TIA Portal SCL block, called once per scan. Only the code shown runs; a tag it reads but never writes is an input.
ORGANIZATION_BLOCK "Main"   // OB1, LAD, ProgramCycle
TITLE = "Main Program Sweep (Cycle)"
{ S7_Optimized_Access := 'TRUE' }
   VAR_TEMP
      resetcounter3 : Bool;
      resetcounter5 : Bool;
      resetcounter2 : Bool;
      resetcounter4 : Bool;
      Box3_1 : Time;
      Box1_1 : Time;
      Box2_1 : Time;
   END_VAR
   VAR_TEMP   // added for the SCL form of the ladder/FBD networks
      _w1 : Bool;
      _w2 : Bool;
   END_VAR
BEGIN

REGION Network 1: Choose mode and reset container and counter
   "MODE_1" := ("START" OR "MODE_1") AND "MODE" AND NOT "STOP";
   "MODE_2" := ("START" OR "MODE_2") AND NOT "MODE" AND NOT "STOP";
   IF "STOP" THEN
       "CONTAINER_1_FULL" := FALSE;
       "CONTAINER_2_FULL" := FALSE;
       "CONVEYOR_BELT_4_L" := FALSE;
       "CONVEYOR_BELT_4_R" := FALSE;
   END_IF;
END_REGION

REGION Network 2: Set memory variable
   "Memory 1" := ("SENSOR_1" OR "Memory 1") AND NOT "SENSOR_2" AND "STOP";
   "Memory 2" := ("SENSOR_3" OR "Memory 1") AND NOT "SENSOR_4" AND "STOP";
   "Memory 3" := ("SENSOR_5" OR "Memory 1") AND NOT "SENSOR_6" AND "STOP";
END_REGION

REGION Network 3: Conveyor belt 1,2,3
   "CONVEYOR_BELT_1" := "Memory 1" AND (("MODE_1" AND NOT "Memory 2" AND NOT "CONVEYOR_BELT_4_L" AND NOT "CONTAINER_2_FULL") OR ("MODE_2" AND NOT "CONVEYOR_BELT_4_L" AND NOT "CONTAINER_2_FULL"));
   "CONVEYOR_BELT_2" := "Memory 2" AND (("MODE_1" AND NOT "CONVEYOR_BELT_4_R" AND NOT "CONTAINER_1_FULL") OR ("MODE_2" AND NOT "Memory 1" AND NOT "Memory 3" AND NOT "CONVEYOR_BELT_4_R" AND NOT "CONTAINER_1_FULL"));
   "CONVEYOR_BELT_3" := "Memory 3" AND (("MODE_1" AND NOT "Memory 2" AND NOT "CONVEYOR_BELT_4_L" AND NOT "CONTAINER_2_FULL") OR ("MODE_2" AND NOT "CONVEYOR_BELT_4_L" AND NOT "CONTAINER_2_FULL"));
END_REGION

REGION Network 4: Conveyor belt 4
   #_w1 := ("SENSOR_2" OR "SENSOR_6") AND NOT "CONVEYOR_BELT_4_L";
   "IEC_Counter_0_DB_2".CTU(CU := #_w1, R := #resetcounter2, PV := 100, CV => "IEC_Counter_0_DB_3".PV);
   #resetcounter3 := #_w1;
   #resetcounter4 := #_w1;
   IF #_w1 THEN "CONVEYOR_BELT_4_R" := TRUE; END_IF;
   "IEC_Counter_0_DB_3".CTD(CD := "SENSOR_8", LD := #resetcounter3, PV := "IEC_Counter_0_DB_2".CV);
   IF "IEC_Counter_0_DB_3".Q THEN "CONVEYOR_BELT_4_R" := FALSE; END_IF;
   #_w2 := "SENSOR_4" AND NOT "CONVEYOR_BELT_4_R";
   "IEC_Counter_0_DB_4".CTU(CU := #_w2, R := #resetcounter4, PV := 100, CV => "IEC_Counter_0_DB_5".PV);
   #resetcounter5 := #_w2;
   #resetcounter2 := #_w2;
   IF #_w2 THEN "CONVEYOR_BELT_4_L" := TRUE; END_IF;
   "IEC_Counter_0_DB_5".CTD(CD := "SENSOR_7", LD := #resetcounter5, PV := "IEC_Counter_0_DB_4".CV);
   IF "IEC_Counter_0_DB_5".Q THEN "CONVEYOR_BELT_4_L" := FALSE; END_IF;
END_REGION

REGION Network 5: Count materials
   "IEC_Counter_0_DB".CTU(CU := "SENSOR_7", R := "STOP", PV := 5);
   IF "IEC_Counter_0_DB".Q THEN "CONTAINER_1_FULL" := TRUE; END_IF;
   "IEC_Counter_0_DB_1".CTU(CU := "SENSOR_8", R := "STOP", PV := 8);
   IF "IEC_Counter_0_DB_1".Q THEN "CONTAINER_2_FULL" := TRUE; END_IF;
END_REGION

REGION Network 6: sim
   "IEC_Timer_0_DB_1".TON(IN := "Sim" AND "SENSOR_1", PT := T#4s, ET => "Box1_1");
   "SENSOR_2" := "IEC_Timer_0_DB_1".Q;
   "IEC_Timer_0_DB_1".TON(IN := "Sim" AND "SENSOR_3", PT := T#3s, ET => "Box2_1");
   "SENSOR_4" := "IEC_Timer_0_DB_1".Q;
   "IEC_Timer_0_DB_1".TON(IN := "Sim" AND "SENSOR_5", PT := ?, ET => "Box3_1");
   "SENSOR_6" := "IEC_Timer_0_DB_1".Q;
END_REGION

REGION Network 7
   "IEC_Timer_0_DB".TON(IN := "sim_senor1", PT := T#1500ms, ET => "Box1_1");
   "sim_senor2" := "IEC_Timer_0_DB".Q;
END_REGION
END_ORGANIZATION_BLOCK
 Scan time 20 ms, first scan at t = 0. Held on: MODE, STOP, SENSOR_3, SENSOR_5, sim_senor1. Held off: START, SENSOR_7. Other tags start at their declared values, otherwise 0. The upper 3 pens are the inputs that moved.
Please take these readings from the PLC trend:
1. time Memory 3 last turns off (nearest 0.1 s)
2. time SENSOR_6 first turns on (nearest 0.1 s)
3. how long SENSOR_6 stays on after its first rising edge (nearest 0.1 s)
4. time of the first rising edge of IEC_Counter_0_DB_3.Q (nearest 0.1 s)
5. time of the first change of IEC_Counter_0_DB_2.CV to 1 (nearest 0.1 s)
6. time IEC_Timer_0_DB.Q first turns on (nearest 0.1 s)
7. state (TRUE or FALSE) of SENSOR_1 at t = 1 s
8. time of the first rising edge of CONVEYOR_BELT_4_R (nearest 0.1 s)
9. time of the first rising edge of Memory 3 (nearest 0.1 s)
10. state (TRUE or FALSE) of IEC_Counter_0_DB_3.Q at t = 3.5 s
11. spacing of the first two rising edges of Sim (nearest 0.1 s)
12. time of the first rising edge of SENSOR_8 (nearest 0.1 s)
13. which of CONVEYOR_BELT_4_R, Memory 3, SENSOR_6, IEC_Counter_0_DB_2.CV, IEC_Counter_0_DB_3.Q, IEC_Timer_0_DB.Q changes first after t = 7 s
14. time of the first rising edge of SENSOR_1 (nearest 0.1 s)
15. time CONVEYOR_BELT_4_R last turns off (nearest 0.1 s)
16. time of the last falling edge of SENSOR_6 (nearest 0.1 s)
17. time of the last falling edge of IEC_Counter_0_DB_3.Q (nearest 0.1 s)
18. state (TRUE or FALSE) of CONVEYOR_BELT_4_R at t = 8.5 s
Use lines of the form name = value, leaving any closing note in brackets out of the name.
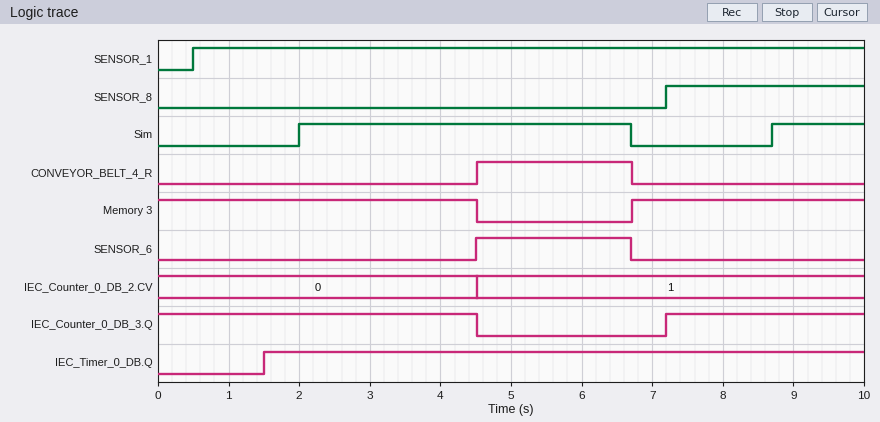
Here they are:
time Memory 3 last turns off = 4.5 s
time SENSOR_6 first turns on = 4.5 s
how long SENSOR_6 stays on after its first rising edge = 2.2 s
time of the first rising edge of IEC_Counter_0_DB_3.Q = 7.2 s
time of the first change of IEC_Counter_0_DB_2.CV to 1 = 4.5 s
time IEC_Timer_0_DB.Q first turns on = 1.5 s
state (TRUE or FALSE) of SENSOR_1 at t = 1 s = TRUE
time of the first rising edge of CONVEYOR_BELT_4_R = 4.5 s
time of the first rising edge of Memory 3 = 6.7 s
state (TRUE or FALSE) of IEC_Counter_0_DB_3.Q at t = 3.5 s = TRUE
spacing of the first two rising edges of Sim = 6.7 s
time of the first rising edge of SENSOR_8 = 7.2 s
which of CONVEYOR_BELT_4_R, Memory 3, SENSOR_6, IEC_Counter_0_DB_2.CV, IEC_Counter_0_DB_3.Q, IEC_Timer_0_DB.Q changes first after t = 7 s = IEC_Counter_0_DB_3.Q
time of the first rising edge of SENSOR_1 = 0.5 s
time CONVEYOR_BELT_4_R last turns off = 6.7 s
time of the last falling edge of SENSOR_6 = 6.7 s
time of the last falling edge of IEC_Counter_0_DB_3.Q = 4.5 s
state (TRUE or FALSE) of CONVEYOR_BELT_4_R at t = 8.5 s = FALSE
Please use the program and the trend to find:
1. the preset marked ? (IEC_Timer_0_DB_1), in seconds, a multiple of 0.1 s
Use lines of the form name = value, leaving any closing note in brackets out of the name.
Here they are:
the preset marked ? (IEC_Timer_0_DB_1), in seconds, a multiple of 0.1 s = 2.5 s
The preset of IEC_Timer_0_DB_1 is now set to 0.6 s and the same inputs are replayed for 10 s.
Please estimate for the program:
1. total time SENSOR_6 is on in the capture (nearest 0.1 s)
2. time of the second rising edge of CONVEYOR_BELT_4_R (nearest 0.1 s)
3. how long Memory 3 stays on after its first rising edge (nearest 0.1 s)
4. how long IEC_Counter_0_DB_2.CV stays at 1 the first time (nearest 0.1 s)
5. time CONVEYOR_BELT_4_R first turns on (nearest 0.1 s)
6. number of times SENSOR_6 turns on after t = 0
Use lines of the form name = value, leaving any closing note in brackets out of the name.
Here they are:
total time SENSOR_6 is on in the capture = 4.8 s
time of the second rising edge of CONVEYOR_BELT_4_R = 9.3 s
how long Memory 3 stays on after its first rising edge = 2.6 s
how long IEC_Counter_0_DB_2.CV stays at 1 the first time = 6.7 s
time CONVEYOR_BELT_4_R first turns on = 2.6 s
number of times SENSOR_6 turns on after t = 0 = 2
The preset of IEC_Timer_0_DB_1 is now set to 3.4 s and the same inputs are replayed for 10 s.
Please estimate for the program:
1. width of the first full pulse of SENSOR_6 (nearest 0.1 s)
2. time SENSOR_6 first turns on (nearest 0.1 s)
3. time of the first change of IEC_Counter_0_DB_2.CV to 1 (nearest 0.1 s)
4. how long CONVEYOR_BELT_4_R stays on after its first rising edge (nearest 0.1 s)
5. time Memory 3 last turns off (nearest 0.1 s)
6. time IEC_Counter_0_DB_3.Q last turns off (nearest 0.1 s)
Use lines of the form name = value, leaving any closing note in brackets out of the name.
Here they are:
width of the first full pulse of SENSOR_6 = 1.7 s
time SENSOR_6 first turns on = 5.0 s
time of the first change of IEC_Counter_0_DB_2.CV to 1 = 5.0 s
how long CONVEYOR_BELT_4_R stays on after its first rising edge = 1.7 s
time Memory 3 last turns off = 5.0 s
time IEC_Counter_0_DB_3.Q last turns off = 5.0 s
